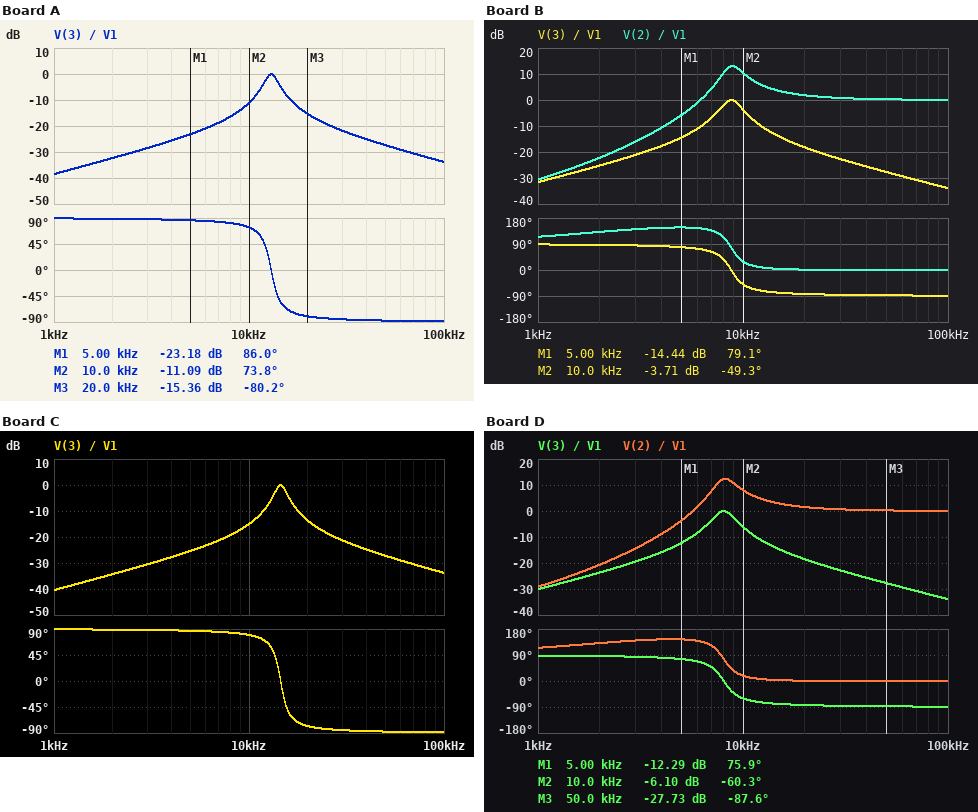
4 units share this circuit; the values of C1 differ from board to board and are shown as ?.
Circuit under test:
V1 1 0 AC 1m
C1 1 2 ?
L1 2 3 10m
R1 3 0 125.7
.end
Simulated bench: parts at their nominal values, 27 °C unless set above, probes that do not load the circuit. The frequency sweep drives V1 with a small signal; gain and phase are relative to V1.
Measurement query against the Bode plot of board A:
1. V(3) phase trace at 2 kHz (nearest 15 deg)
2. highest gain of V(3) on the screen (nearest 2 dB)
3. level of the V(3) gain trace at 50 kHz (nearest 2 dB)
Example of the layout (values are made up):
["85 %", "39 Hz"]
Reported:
["90 deg", "0 dB", "-28 dB"]
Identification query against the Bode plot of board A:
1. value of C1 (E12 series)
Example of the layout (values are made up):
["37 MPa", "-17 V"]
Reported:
["15 nF"]
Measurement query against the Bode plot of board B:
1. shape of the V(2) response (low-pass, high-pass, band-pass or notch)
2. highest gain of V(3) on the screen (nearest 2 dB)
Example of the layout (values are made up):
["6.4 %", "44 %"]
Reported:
["high-pass", "0 dB"]
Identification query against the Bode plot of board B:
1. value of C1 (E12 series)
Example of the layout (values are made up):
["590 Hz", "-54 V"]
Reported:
["33 nF"]
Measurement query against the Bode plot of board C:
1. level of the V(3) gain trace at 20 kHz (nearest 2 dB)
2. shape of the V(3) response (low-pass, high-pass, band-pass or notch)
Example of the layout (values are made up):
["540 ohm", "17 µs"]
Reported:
["-14 dB", "band-pass"]
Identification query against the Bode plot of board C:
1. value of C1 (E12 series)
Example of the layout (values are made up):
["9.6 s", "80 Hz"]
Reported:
["12 nF"]
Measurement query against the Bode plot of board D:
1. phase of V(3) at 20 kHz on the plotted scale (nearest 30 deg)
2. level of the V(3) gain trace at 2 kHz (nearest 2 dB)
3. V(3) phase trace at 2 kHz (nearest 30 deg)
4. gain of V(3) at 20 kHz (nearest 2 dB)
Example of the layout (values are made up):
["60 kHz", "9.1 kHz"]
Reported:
["-90 deg", "-24 dB", "90 deg", "-18 dB"]
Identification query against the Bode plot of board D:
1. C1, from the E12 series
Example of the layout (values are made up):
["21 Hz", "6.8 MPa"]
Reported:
["39 nF"]
